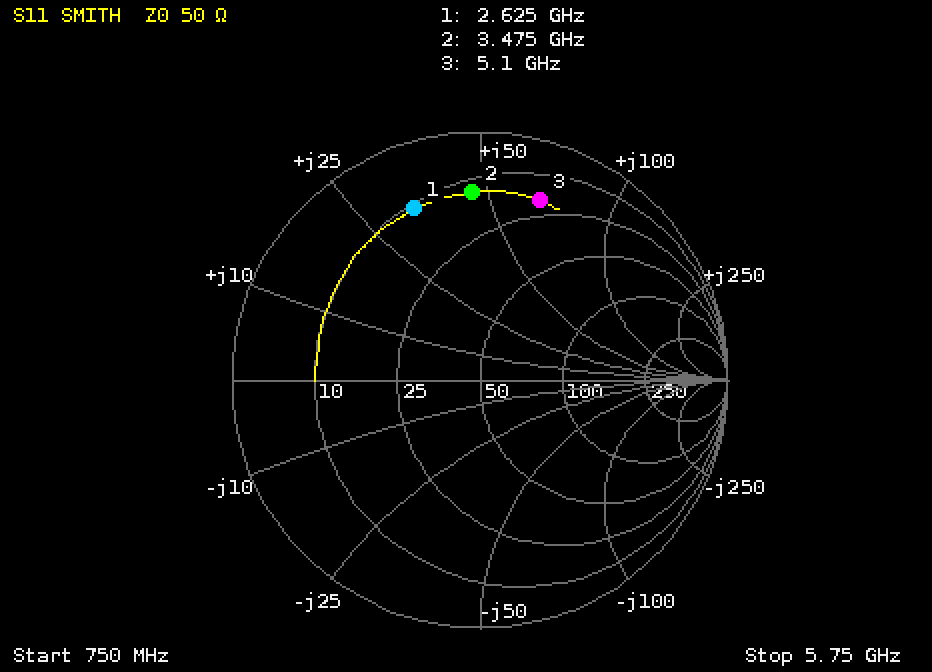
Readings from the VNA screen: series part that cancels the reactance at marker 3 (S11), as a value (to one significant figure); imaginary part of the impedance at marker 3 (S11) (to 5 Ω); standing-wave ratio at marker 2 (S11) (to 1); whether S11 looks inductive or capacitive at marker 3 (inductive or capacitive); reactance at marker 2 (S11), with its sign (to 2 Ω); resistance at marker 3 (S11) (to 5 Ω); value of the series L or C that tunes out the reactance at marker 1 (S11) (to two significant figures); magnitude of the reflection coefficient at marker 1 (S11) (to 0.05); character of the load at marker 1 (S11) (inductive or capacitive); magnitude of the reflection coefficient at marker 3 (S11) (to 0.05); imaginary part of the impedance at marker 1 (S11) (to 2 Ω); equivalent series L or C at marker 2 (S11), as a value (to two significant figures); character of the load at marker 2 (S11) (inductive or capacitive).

500 fF
+65 Ω
7
inductive
+46 Ω
20 Ω
1.8 pF
0.75
inductive
0.75
+34 Ω
2.1 nH
inductive
